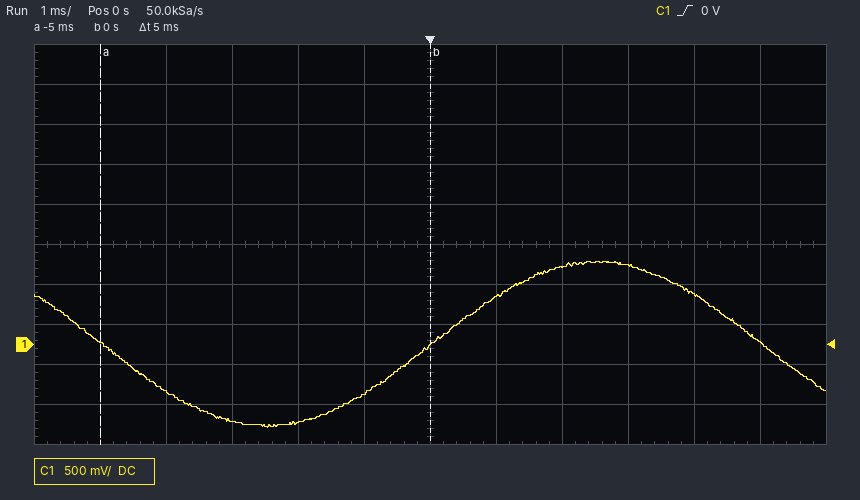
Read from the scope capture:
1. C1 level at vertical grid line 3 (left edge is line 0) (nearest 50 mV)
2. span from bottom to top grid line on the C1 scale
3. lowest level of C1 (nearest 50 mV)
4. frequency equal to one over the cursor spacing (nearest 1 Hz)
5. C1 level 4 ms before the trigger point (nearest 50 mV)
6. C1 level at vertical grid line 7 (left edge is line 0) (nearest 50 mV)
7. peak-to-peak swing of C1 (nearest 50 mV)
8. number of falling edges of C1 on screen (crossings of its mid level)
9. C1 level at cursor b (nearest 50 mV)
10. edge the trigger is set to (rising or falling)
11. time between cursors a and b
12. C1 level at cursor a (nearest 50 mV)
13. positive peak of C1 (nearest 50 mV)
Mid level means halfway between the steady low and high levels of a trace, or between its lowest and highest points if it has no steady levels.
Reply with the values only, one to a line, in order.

-950 mV
5 V
-1.05 V
200 Hz
-600 mV
600 mV
2.10 V
2
0 mV
rising
5 ms
0 mV
1.05 V
